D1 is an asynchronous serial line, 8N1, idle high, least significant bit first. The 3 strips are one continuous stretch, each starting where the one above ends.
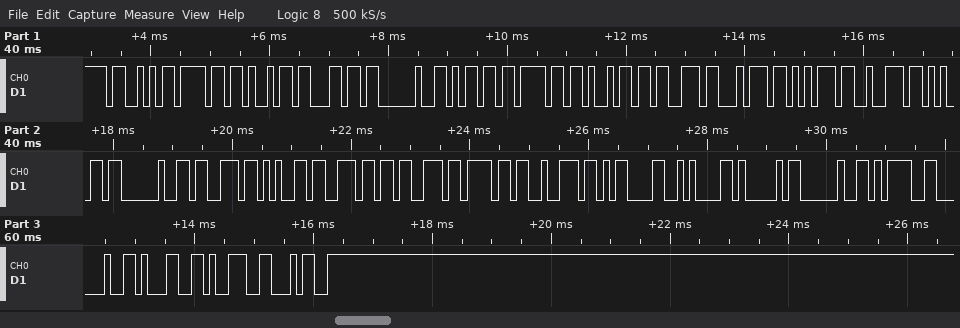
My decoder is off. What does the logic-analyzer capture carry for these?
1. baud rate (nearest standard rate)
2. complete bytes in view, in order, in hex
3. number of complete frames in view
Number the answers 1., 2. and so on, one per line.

1. 9600 baud
2. 0x53 0x6F 0x69 0x6C 0x20 0x6D 0x6F 0x69 0x73 0x74 0x75 0x72 0x65 0x20 0x73 0x65 0x6E 0x73 0x6F 0x72 0x0D 0x0A 0x41 0x20 0x3D 0x20 0x31 0x39 0x34
3. 29
